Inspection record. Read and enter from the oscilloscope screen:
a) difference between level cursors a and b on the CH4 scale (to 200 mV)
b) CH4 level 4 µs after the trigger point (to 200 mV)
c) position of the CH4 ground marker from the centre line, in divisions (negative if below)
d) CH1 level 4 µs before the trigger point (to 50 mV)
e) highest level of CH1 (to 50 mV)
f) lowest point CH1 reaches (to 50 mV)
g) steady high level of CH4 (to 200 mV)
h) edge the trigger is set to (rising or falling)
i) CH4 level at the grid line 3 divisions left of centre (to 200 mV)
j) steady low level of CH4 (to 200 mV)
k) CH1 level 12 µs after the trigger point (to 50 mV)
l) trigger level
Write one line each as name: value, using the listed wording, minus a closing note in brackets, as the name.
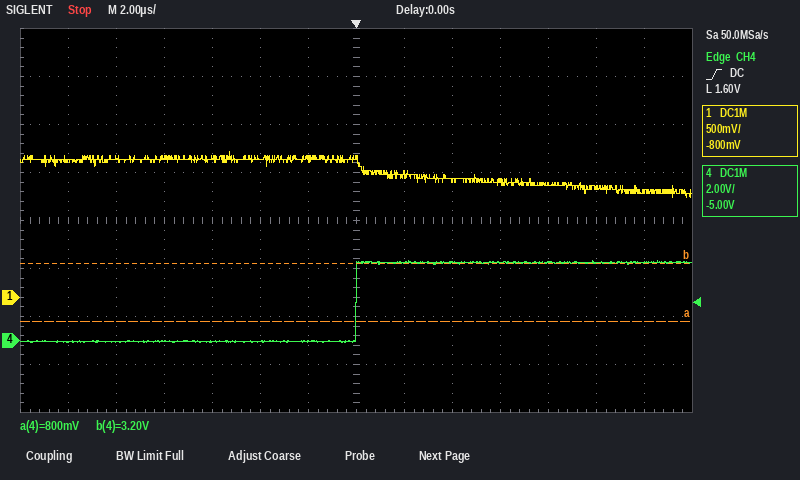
difference between level cursors a and b on the CH4 scale: 2.4 V
CH4 level 4 µs after the trigger point: 3.2 V
position of the CH4 ground marker from the centre line, in divisions: -2.5 div
CH1 level 4 µs before the trigger point: 1.45 V
highest level of CH1: 1.50 V
lowest point CH1 reaches: 1.05 V
steady high level of CH4: 3.2 V
edge the trigger is set to: rising
CH4 level at the grid line 3 divisions left of centre: 0.0 V
steady low level of CH4: 0.0 V
CH1 level 12 µs after the trigger point: 1.10 V
trigger level: 1.60 V
